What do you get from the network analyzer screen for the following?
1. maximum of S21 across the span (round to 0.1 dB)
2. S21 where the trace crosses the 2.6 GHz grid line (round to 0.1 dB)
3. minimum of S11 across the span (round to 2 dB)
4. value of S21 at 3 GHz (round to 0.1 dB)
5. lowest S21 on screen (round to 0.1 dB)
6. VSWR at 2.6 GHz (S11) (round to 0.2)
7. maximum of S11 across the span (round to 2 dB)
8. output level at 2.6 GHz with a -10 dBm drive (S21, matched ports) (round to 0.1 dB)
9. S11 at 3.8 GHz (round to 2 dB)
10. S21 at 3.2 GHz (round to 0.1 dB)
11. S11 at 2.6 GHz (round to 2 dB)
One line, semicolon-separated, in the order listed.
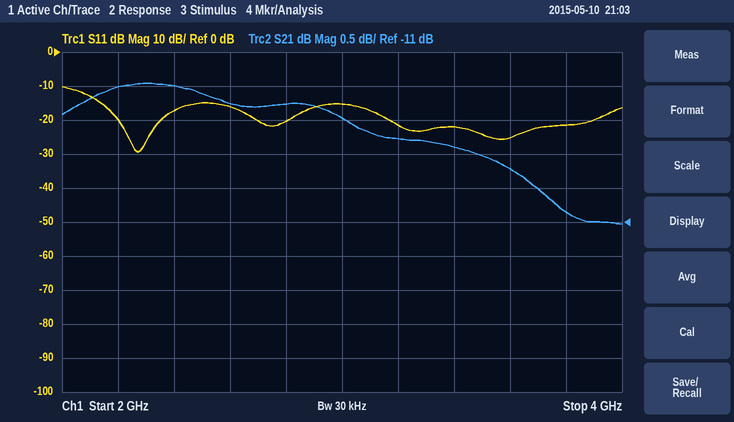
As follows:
-9.0 dB; -9.3 dB; -30 dB; -9.5 dB; -11.0 dB; 1.4; -10 dB; -19.3 dBm; -22 dB; -9.8 dB; -16 dB
